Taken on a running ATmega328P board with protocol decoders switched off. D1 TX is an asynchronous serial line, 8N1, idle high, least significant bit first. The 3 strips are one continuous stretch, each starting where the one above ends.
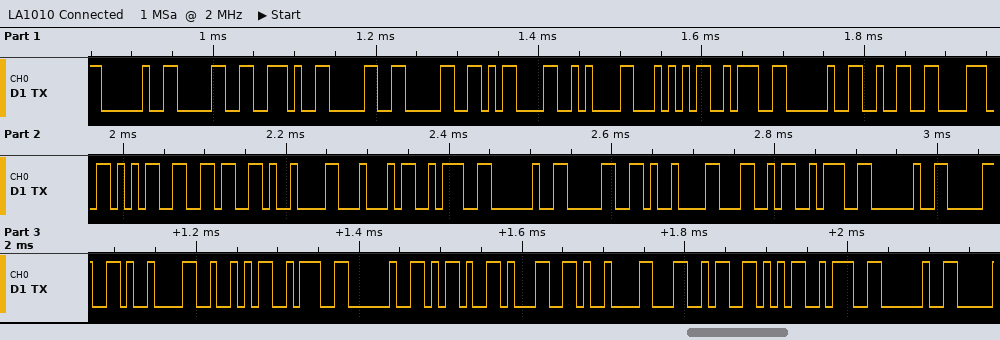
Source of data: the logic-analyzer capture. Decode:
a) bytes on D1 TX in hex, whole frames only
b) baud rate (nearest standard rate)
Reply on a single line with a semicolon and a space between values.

0x20 0x30 0x2E 0x30 0x30 0x0D 0x0A 0x54 0x3A 0x20 0x32 0x38 0x35 0x36 0x09 0x44 0x3A 0x20 0x30 0x09 0x4C 0x3A 0x20 0x30 0x09 0x52 0x3A 0x20 0x2D 0x31 0x09 0x4C 0x56 0x3A 0x20; 115200 baud
